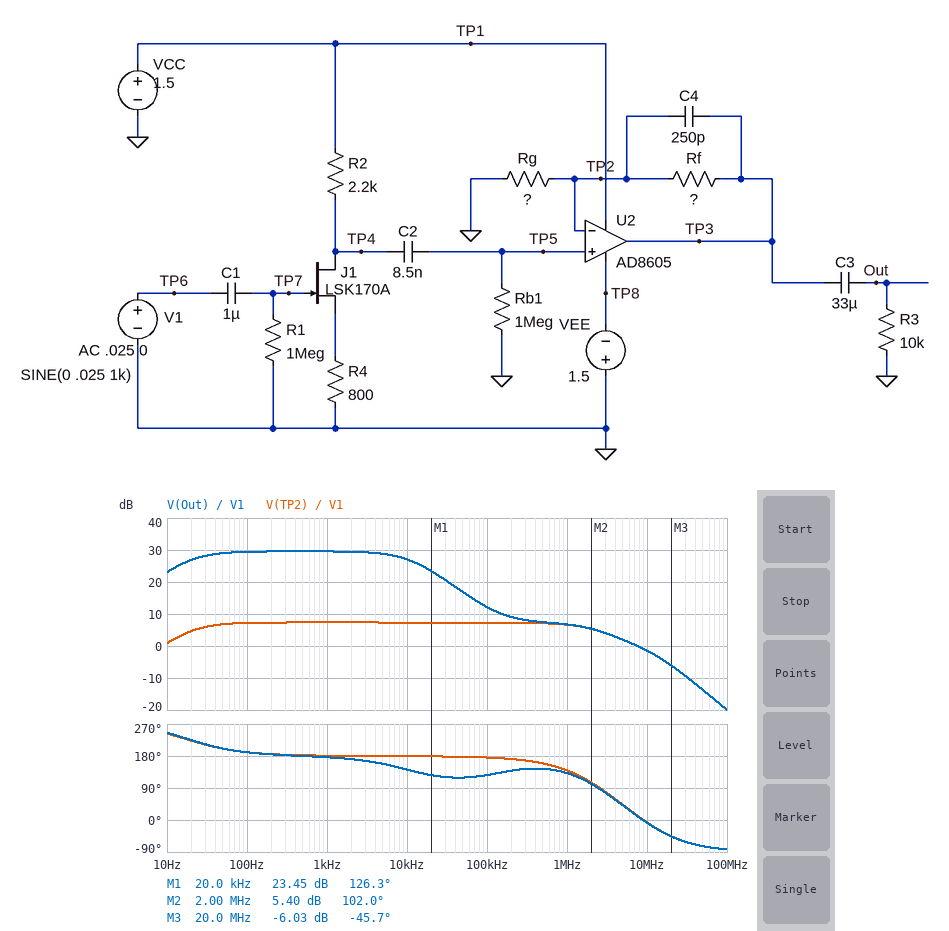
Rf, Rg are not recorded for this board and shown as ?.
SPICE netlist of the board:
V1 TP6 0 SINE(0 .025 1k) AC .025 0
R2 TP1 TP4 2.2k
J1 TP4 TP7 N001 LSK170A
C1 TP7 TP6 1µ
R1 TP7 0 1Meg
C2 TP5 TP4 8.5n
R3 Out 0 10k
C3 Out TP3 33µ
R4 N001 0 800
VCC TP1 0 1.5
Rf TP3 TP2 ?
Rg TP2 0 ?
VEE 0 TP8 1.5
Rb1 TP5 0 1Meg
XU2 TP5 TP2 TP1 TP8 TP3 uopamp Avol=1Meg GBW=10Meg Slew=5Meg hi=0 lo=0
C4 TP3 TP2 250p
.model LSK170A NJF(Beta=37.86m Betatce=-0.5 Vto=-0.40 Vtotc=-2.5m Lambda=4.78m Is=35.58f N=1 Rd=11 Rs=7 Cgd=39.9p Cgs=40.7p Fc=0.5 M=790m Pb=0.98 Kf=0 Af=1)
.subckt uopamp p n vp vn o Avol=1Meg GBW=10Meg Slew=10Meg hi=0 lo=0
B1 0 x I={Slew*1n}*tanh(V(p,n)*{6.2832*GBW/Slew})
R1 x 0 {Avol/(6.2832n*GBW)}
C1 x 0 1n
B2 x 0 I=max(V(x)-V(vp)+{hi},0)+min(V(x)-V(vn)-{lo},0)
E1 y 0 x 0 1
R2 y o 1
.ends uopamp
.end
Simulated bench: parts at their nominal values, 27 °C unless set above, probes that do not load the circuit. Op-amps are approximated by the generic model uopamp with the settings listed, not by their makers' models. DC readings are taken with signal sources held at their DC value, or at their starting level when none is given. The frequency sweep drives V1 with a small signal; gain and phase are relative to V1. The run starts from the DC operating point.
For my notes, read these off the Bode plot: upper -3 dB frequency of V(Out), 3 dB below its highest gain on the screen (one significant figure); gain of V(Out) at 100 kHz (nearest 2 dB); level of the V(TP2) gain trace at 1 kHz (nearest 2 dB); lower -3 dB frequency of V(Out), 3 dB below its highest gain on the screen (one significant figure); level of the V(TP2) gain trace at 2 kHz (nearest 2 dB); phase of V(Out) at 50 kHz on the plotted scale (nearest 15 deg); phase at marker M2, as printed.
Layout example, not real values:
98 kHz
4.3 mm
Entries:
10 kHz
12 dB
8 dB
20 Hz
8 dB
120 deg
102.0 deg
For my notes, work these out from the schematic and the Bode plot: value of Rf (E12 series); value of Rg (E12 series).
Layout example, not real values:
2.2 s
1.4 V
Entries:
56 kΩ
4.7 kΩ
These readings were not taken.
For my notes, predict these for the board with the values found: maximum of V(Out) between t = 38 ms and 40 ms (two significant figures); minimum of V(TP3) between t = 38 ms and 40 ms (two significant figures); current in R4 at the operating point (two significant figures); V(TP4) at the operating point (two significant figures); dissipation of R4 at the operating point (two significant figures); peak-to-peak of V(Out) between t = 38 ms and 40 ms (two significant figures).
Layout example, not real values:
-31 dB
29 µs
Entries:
750 mV
-750 mV
370 µA
680 mV
110 µW
1.5 V
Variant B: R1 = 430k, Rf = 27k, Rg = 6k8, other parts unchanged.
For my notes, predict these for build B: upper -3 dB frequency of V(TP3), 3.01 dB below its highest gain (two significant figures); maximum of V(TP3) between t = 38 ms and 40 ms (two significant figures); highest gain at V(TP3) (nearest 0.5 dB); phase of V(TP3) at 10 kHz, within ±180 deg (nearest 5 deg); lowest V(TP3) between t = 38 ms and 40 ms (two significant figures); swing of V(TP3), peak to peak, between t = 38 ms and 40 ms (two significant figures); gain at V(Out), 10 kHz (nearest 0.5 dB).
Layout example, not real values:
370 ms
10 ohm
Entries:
24 kHz
290 mV
21.5 dB
160 deg
-290 mV
580 mV
20.5 dB
